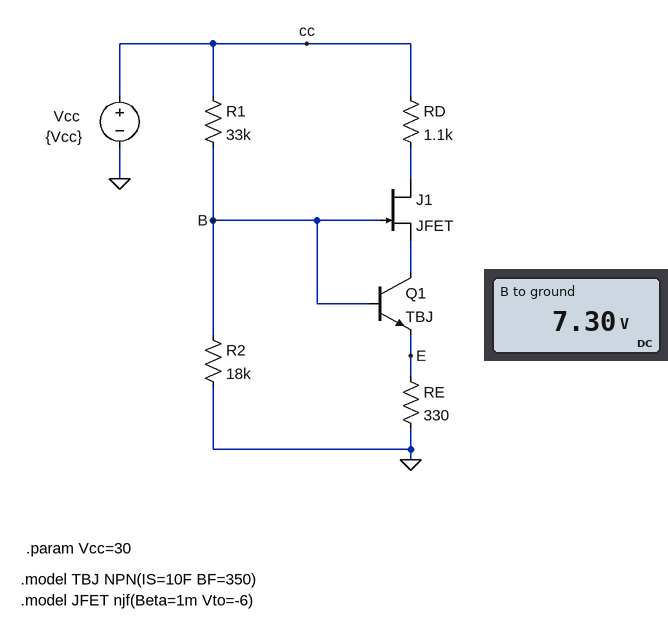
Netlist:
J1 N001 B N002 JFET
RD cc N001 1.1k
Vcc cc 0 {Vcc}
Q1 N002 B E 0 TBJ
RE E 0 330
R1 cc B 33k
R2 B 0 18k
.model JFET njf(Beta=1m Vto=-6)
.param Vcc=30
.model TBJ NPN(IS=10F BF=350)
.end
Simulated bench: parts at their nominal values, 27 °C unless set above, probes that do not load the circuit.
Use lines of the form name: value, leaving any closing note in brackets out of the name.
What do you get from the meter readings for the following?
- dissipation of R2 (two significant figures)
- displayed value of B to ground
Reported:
dissipation of R2: 3.0 mW
displayed value of B to ground: 7.30 V
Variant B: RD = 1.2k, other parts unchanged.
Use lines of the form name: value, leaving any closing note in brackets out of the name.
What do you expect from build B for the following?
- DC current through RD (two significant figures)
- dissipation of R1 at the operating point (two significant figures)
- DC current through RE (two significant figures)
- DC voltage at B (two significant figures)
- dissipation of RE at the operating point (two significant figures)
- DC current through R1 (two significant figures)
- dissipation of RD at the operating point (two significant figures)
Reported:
DC current through RD: 18 mA
dissipation of R1 at the operating point: 16 mW
DC current through RE: 19 mA
DC voltage at B: 6.9 V
dissipation of RE at the operating point: 120 mW
DC current through R1: 700 µA
dissipation of RD at the operating point: 410 mW
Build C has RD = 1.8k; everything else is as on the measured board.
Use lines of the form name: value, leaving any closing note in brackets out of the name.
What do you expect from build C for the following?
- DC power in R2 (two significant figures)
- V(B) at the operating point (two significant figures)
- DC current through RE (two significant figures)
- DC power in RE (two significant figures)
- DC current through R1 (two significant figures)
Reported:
DC power in R2: 1.6 mW
V(B) at the operating point: 5.3 V
DC current through RE: 14 mA
DC power in RE: 64 mW
DC current through R1: 750 µA
